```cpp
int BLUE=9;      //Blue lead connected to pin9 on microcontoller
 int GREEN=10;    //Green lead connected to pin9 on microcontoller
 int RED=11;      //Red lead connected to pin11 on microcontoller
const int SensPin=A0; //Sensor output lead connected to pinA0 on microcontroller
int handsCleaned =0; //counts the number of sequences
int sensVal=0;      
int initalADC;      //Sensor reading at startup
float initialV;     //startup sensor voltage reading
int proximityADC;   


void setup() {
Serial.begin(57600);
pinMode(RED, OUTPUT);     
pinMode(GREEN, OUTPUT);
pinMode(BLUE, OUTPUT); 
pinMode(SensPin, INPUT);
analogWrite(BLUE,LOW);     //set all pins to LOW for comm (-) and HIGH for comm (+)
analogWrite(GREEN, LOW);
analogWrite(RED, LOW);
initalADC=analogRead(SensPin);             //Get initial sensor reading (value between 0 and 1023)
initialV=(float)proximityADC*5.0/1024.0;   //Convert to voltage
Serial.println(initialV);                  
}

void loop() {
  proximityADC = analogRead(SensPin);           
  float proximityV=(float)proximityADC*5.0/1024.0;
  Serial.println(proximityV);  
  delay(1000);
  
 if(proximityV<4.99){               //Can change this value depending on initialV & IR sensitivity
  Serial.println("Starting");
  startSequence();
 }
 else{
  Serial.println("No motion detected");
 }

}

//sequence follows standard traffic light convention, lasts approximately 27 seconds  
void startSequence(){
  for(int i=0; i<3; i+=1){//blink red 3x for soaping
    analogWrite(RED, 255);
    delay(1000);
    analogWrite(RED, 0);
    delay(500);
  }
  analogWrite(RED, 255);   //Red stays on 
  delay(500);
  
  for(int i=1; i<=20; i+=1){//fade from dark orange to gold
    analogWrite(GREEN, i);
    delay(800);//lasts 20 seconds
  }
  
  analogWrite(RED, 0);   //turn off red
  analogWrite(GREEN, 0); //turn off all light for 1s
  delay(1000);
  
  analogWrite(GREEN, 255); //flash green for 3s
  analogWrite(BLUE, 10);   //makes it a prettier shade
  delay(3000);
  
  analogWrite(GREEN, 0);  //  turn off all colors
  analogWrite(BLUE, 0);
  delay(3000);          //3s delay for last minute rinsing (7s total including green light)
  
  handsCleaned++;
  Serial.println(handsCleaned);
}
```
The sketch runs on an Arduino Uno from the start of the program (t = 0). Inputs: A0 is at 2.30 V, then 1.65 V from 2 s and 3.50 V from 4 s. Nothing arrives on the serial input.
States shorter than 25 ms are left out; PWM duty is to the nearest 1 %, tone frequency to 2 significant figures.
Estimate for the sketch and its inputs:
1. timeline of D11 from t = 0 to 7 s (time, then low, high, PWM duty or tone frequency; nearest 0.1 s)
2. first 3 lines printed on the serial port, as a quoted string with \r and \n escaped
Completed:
0 s low; 1 s high; 2 s low; 2.5 s high; 3.5 s low; 4 s high; 5 s low; 5.5 s high
"0.00\r\n2.30\r\nStarting\r\n"
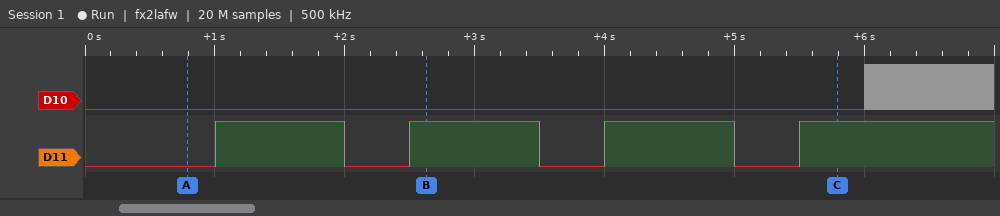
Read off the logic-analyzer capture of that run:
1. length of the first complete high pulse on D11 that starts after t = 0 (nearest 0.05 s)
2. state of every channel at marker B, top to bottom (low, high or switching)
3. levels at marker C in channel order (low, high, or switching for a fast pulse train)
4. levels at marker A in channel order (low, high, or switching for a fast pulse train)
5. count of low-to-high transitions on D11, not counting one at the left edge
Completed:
1.00 s
D10 low, D11 high
D10 low, D11 high
D10 low, D11 low
4
